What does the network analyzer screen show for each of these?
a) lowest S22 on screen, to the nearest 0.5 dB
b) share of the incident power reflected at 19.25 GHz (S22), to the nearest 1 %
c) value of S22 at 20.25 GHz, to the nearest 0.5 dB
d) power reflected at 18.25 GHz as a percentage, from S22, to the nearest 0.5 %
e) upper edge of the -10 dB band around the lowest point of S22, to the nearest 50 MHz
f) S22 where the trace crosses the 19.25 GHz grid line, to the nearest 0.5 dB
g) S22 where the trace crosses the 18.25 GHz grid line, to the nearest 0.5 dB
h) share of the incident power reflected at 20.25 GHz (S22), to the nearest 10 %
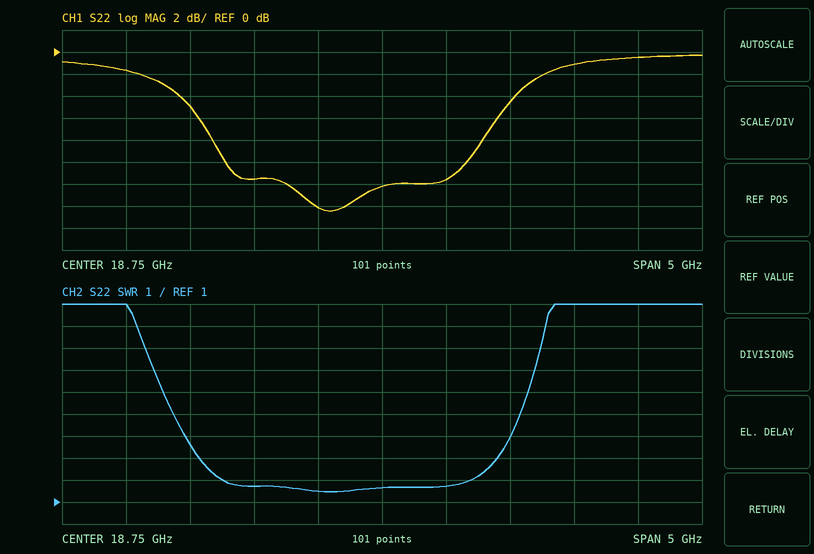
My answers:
-14.5 dB
7 %
-1.0 dB
4.0 %
19.40 GHz
-11.5 dB
-14.0 dB
80 %
